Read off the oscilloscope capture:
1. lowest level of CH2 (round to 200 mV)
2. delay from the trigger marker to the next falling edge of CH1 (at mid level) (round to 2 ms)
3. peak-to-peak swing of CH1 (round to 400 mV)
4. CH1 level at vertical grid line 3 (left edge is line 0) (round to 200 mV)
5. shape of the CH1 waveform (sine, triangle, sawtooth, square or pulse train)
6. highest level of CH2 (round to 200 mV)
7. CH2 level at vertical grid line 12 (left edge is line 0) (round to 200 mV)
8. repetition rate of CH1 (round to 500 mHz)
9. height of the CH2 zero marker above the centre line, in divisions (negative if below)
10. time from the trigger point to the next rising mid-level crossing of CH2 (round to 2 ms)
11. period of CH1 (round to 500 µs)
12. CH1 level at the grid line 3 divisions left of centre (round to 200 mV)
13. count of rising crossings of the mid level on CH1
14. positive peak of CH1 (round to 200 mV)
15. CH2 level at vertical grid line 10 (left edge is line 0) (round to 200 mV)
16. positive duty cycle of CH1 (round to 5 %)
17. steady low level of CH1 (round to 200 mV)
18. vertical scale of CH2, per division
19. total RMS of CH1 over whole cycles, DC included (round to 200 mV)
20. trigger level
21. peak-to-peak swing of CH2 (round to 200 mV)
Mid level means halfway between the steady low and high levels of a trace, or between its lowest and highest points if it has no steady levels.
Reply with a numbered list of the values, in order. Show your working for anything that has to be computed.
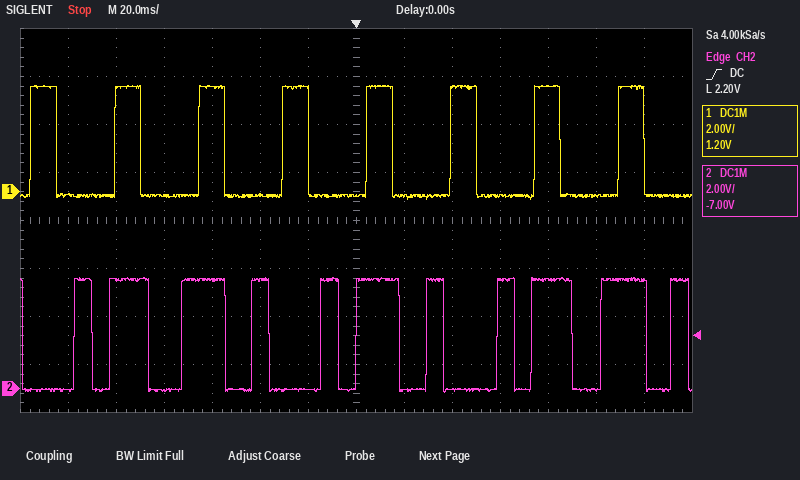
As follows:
1. -200 mV
2. 16 ms
3. 4.8 V
4. -200 mV
5. pulse train
6. 4.6 V
7. 0.0 V
8. 1 / 35.0 ms ≈ 28.6 Hz, so 28.5 Hz to the nearest 500 mHz
9. -3.5 div
10. 30 ms
11. 35.0 ms
12. 4.4 V
13. 8
14. 4.4 V
15. 4.6 V
16. 30 %
17. -200 mV
18. 2 V
19. √(0.3 × (4.4 V)² + 0.7 × (-200 mV)²) ≈ 2.4 V
20. 2.20 V
21. 4.6 V − (-200 mV) = 4.8 V
